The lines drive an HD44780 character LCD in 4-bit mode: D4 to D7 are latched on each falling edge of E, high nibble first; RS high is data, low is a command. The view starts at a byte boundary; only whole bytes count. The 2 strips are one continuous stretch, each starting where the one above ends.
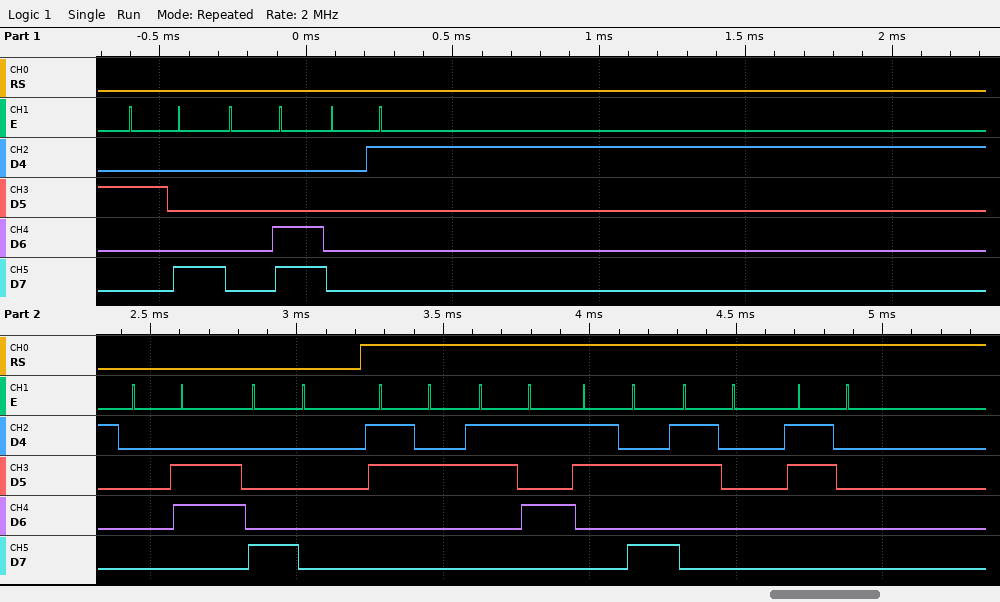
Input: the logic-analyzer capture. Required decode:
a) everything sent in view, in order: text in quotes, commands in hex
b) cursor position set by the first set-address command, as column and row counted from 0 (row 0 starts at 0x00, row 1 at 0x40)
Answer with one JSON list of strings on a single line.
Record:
["0x28 0x0C 0x01 0x06 0x80 \"25:00\"", "column 0, row 0"]
